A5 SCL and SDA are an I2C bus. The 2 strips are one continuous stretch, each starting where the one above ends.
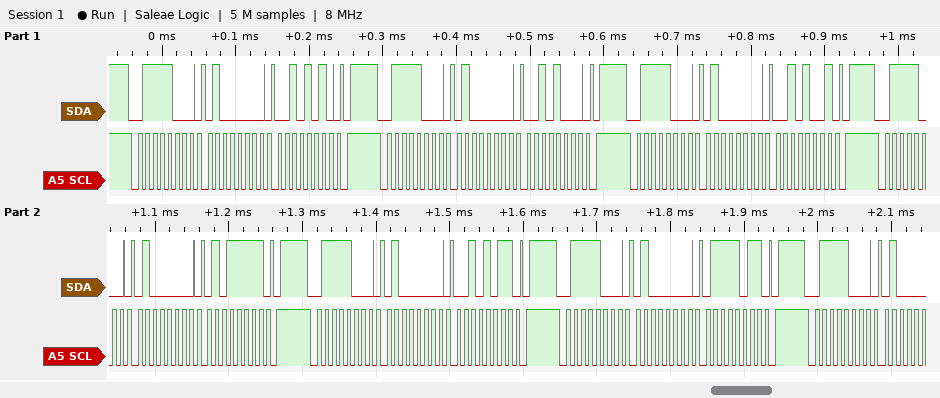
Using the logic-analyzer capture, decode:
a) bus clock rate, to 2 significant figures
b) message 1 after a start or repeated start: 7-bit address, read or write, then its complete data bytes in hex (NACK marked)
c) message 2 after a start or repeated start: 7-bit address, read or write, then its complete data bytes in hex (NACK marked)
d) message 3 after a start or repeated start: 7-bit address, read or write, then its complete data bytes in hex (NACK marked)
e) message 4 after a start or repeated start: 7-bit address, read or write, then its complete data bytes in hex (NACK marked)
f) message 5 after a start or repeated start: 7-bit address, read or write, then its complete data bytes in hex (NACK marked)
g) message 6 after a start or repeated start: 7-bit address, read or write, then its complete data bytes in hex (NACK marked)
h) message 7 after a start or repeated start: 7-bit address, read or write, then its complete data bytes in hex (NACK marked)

100 kHz
0x3C write: 40 2A
0x3C write: 40 28
0x3C write: 40 29
0x3C write: 40 5F
0x3C write: 40 2B
0x3C write: 40 7B
0x3C write
